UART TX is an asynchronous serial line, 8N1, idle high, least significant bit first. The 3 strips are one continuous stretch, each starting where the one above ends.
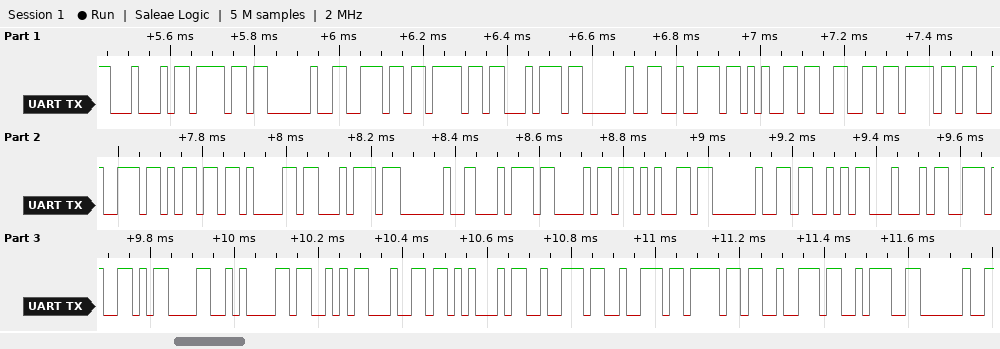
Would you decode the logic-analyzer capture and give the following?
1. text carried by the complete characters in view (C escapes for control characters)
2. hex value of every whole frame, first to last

"Do not reformat the SD.\r\nSdError: "
44 6F 20 6E 6F 74 20 72 65 66 6F 72 6D 61 74 20 74 68 65 20 53 44 2E 0D 0A 53 64 45 72 72 6F 72 3A 20
